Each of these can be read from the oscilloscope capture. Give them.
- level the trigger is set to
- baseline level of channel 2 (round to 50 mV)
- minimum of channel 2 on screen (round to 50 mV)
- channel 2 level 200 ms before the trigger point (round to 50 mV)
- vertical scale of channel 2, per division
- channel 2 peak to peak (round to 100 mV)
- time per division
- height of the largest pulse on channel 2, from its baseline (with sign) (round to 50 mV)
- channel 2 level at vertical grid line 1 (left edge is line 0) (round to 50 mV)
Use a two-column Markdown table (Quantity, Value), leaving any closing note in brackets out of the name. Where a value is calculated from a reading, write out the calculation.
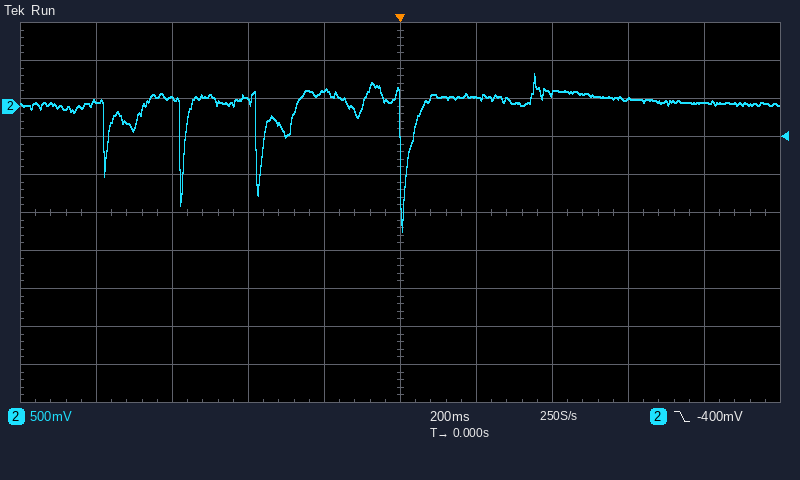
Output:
| Quantity | Value |
|---|---|
| level the trigger is set to | -400 mV |
| baseline level of channel 2 | 50 mV |
| minimum of channel 2 on screen | -1.65 V |
| channel 2 level 200 ms before the trigger point | 200 mV |
| vertical scale of channel 2, per division | 500 mV |
| channel 2 peak to peak | 2.10 V |
| time per division | 200 ms |
| height of the largest pulse on channel 2, from its baseline (with sign) | -1.65 V − (50 mV) = -1.70 V |
| channel 2 level at vertical grid line 1 (left edge is line 0) | 50 mV |
